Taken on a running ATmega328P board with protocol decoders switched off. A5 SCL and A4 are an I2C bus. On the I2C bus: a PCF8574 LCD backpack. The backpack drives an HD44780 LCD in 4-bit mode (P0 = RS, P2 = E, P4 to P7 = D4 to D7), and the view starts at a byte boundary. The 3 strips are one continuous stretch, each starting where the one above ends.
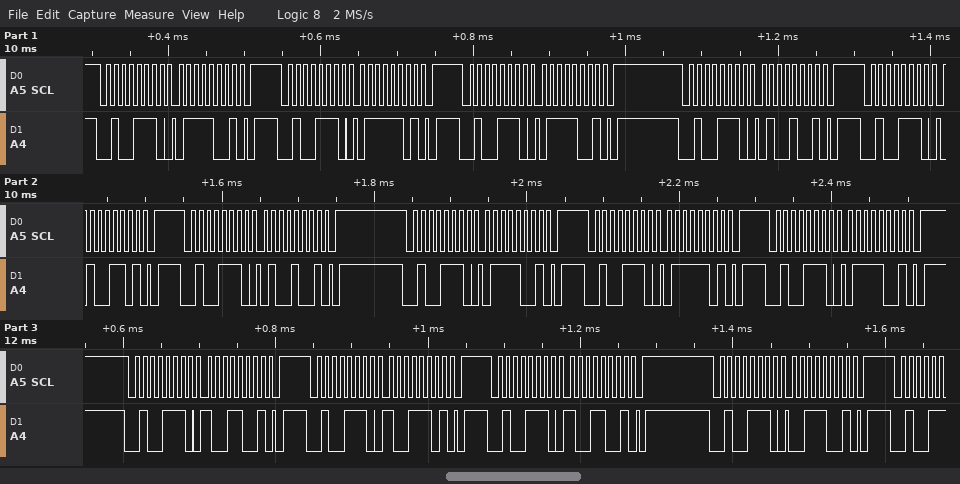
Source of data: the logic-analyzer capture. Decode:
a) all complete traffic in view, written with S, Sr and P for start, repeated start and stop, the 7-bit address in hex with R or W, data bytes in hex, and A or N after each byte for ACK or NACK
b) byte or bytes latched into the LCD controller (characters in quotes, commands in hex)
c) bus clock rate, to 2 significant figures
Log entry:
S 27W A 79 A P S 27W A 7D A P S 27W A 79 A P S 27W A 49 A P S 27W A 4D A P S 27W A 49 A P S 27W A 79 A P S 27W A 7D A P S 27W A 79 A P S 27W A 99 A P S 27W A 9D A P S 27W A 99 A P S 27W A 39 A P
't' 'y'
100 kHz
